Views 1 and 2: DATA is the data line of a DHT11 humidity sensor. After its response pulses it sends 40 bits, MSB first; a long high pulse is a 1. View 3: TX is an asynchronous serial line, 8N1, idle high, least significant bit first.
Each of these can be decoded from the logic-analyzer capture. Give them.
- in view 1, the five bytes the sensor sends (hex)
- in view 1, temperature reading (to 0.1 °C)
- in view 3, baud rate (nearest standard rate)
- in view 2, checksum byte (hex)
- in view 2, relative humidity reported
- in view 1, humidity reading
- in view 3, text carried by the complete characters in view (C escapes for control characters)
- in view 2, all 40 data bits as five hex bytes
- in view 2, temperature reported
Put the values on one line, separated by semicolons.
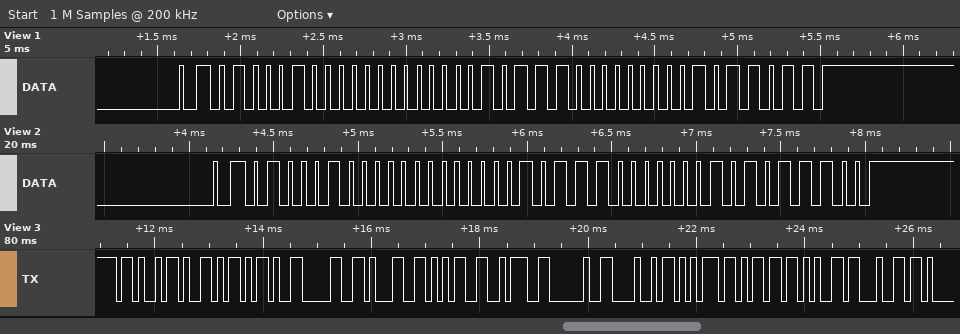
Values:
44 00 17 00 5B; 23.0 °C; 9600 baud; 0x5C; 68 %; 68 %; "KY-015: Humed"; 44 00 17 01 5C; 23.1 °C
